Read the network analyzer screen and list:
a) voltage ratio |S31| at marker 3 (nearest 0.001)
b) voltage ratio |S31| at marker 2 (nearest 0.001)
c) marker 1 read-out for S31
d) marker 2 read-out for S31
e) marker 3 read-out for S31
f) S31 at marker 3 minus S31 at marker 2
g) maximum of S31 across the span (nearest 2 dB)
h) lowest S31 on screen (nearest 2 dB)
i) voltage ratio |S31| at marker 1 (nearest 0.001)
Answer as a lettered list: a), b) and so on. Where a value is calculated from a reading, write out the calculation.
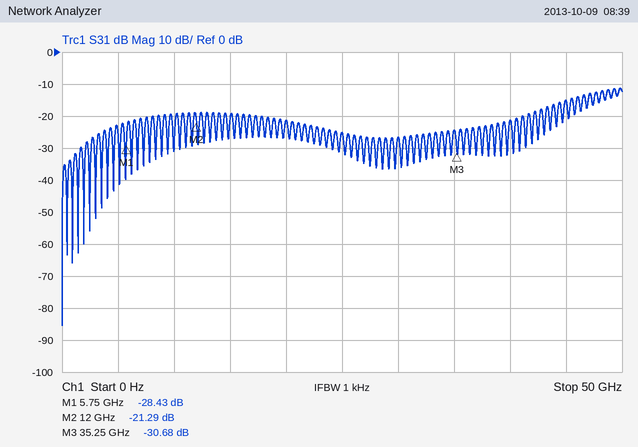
a) 10^(-30.68/20) ≈ 0.029
b) 10^(-21.29/20) ≈ 0.086
c) -28.43 dB
d) -21.29 dB
e) -30.68 dB
f) -30.68 − (-21.29) = -9.39 dB
g) -12 dB
h) -86 dB
i) 10^(-28.43/20) ≈ 0.038
